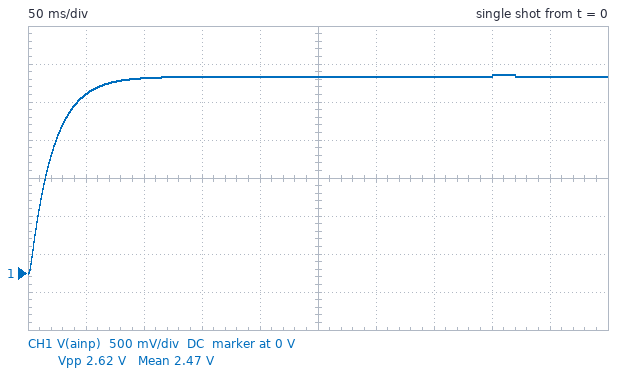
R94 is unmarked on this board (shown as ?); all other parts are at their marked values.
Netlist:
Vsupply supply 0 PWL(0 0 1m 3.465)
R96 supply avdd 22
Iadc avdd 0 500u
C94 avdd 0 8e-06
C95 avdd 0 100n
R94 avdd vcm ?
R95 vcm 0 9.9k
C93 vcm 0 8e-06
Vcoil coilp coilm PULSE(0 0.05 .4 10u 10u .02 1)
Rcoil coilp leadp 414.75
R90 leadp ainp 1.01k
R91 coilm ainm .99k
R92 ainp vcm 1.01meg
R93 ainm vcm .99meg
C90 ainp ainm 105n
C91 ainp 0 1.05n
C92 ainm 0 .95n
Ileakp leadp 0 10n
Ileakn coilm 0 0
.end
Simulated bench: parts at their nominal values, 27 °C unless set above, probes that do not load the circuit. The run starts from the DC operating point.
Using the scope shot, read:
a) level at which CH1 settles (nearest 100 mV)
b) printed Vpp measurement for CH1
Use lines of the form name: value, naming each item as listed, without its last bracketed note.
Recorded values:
level at which CH1 settles: 2.6 V
printed Vpp measurement for CH1: 2.62 V
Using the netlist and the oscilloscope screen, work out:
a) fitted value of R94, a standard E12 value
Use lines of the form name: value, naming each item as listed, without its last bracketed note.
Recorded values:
fitted value of R94, a standard E12 value: 3.3 kΩ
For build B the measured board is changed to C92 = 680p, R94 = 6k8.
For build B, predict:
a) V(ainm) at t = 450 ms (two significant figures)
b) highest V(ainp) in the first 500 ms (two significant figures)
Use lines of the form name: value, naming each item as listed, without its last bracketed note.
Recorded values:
V(ainm) at t = 450 ms: 2.0 V
highest V(ainp) in the first 500 ms: 2.1 V
